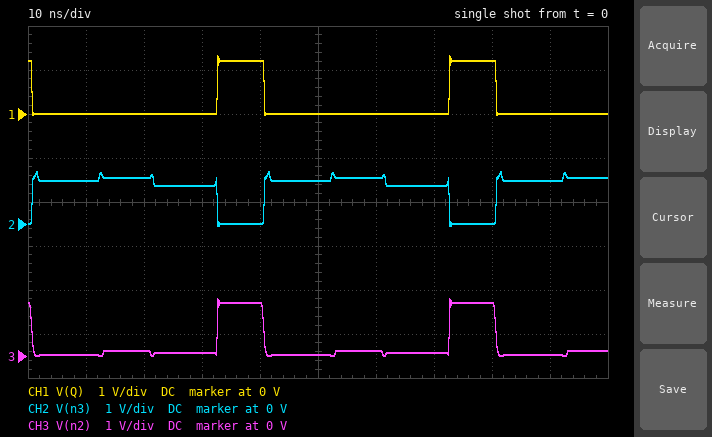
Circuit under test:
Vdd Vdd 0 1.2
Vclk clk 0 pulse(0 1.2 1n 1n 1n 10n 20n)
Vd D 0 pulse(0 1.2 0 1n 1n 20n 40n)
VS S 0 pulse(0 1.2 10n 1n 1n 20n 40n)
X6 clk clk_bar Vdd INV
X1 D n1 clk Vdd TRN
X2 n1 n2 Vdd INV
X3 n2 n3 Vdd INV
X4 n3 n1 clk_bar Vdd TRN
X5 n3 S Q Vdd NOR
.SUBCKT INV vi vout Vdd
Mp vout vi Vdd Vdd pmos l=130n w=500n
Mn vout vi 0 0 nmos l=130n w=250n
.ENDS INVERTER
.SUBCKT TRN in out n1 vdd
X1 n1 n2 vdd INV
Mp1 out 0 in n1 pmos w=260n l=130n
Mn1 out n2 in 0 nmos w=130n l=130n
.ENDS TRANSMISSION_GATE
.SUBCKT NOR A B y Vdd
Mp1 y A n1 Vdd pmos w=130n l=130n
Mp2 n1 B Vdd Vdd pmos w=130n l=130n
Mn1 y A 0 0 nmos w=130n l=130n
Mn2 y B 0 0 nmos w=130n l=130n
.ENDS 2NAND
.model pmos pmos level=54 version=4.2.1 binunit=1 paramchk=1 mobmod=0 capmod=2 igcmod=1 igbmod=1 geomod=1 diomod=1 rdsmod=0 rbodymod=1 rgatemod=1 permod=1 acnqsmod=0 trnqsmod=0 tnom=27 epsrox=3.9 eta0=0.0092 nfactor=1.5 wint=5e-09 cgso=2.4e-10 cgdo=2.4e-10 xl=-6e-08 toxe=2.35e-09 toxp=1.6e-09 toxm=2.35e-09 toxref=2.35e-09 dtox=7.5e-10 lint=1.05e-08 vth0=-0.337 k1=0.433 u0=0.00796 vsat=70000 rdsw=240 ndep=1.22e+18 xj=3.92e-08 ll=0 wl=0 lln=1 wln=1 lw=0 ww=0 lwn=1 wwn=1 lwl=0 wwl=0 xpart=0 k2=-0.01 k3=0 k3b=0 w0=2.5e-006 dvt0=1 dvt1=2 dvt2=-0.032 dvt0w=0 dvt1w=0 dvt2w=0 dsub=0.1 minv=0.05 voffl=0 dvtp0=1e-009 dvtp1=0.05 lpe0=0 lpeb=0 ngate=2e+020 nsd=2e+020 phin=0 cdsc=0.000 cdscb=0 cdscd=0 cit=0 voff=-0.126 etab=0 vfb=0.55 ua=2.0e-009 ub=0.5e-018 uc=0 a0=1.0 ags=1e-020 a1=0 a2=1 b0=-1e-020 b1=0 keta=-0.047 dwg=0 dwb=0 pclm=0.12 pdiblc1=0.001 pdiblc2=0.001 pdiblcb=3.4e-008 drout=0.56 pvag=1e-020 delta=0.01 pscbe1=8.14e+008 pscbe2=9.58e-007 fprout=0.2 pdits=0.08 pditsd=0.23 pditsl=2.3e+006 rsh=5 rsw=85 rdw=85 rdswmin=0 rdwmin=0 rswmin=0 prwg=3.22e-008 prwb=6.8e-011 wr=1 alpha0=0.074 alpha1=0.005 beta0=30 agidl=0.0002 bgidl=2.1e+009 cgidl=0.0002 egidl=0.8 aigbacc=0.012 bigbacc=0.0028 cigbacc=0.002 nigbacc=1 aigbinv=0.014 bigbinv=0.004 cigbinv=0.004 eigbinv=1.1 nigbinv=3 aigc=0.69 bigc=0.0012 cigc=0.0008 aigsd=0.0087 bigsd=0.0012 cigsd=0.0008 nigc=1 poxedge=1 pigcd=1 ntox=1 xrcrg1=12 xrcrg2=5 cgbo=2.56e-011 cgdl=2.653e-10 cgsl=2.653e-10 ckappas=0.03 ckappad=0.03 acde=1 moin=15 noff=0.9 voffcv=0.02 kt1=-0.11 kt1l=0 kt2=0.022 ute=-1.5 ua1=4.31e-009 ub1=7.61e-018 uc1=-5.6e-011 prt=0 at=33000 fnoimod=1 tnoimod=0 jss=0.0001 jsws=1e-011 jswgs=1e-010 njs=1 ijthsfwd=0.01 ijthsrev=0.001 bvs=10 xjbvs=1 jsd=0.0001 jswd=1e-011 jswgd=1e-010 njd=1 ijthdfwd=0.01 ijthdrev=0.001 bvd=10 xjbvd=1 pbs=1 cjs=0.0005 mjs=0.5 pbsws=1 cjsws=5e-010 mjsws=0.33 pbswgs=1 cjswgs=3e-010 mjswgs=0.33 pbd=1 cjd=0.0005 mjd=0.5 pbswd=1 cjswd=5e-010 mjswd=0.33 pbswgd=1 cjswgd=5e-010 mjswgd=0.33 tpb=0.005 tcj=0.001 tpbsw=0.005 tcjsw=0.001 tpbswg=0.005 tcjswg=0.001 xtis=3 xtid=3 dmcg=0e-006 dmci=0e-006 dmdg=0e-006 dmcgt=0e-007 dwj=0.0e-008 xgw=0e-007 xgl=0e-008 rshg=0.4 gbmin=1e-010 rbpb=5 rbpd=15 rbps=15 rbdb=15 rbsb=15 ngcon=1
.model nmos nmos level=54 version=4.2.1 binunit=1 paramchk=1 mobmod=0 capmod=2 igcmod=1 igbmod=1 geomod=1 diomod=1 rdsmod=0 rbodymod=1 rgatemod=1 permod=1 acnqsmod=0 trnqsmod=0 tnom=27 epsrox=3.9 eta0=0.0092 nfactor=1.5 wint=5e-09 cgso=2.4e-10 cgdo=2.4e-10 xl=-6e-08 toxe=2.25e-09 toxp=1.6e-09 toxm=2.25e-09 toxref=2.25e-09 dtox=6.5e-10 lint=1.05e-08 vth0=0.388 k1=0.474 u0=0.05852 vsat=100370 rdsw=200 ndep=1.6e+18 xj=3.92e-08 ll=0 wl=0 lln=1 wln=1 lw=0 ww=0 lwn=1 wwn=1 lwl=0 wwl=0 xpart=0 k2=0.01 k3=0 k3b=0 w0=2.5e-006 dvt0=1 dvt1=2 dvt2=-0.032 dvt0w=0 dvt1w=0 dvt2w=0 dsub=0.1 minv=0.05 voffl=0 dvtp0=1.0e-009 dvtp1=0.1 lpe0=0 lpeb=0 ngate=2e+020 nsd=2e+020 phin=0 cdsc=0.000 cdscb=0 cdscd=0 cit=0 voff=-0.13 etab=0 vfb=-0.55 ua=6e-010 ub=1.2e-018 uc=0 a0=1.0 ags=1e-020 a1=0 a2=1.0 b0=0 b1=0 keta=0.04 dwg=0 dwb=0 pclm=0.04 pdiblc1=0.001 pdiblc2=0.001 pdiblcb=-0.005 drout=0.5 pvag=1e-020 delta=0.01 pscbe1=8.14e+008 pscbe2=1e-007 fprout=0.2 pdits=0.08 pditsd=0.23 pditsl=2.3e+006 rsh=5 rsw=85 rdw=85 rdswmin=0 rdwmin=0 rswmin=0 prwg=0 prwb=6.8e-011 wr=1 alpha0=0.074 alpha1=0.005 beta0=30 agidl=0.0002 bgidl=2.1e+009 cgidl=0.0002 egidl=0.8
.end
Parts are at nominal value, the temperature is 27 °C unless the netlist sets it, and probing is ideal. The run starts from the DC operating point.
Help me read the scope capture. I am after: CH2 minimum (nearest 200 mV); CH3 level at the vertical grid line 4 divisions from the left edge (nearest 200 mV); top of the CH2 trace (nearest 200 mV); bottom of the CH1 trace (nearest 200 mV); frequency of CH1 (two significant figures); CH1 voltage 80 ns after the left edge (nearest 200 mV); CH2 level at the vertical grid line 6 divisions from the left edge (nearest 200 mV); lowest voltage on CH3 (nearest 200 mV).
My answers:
0 V
1.2 V
1.2 V
0 V
25 MHz
1.2 V
1.0 V
0 V
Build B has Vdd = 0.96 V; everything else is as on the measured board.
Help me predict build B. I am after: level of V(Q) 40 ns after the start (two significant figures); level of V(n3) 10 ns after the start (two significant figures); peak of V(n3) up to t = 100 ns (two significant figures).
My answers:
960 mV
850 mV
1.0 V
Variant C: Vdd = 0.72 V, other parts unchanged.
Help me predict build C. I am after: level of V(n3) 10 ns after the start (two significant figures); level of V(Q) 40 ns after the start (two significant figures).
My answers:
710 mV
720 mV
